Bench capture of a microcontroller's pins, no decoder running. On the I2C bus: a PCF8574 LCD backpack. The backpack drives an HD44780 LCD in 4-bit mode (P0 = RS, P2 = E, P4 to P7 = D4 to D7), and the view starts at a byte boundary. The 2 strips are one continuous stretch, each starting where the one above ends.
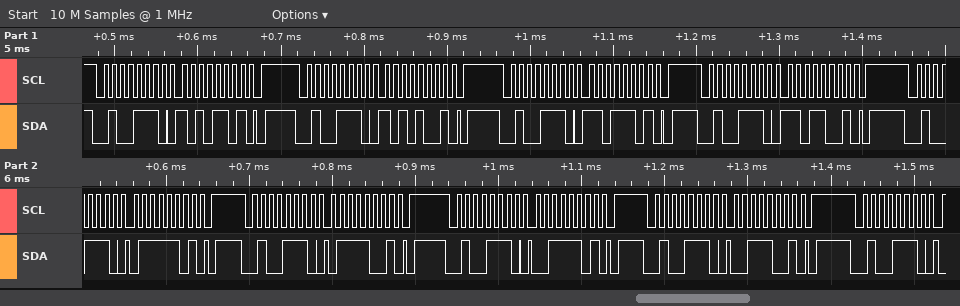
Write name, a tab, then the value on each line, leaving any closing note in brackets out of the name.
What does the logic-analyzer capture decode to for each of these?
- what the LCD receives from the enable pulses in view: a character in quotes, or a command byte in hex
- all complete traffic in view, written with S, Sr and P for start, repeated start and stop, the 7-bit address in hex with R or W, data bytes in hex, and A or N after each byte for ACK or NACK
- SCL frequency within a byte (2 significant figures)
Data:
what the LCD receives from the enable pulses in view: a character in quotes, or a command byte in hex	data 0xAD 's'
all complete traffic in view, written with S, Sr and P for start, repeated start and stop, the 7-bit address in hex with R or W, data bytes in hex, and A or N after each byte for ACK or NACK	S 27W A AD A P S 27W A A9 A P S 27W A DD A P S 27W A D9 A P S 27W A 7D A P S 27W A 79 A P S 27W A 3D A P S 27W A 39 A P S 27W A
SCL frequency within a byte	100 kHz
